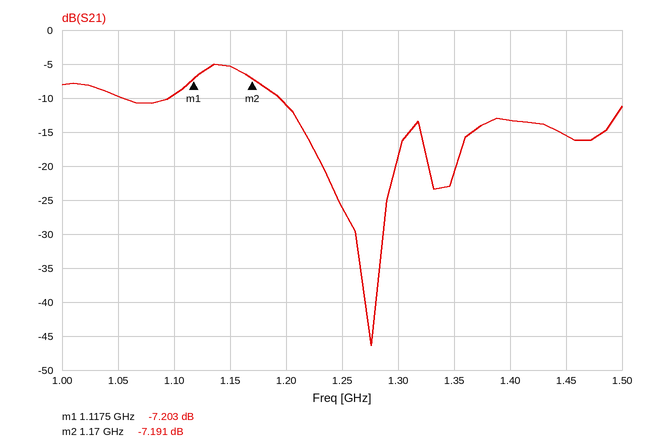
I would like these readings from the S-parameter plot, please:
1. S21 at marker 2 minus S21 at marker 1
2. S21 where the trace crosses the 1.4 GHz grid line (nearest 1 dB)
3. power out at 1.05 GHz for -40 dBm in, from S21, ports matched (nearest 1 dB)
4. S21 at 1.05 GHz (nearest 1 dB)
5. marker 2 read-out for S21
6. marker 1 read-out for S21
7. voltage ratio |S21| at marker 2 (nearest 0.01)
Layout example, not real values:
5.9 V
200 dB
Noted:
0.012 dB
-13 dB
-50 dBm
-10 dB
-7.191 dB
-7.203 dB
0.44
